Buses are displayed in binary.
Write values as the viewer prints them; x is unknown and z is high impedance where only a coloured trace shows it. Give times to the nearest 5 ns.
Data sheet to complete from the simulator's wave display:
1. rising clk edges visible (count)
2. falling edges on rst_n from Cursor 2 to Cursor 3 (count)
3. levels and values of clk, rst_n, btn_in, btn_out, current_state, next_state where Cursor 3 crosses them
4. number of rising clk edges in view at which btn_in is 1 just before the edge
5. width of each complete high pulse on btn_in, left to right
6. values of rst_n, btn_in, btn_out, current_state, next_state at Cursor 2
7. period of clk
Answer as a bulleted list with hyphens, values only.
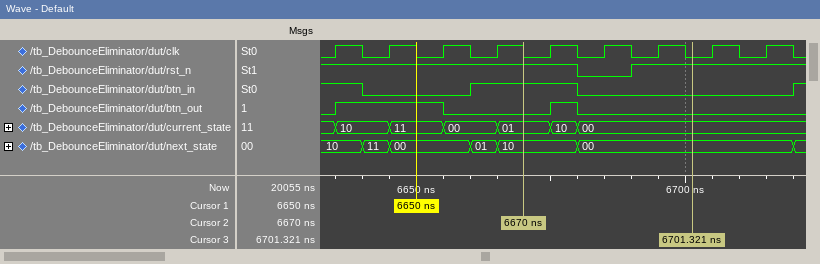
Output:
- 9
- 1
- clk=0, rst_n=1, btn_in=0, btn_out=0, current_state=00, next_state=00
- 3
- 20 ns
- rst_n=1, btn_in=1, btn_out=0, current_state=01, next_state=10
- 10 ns
